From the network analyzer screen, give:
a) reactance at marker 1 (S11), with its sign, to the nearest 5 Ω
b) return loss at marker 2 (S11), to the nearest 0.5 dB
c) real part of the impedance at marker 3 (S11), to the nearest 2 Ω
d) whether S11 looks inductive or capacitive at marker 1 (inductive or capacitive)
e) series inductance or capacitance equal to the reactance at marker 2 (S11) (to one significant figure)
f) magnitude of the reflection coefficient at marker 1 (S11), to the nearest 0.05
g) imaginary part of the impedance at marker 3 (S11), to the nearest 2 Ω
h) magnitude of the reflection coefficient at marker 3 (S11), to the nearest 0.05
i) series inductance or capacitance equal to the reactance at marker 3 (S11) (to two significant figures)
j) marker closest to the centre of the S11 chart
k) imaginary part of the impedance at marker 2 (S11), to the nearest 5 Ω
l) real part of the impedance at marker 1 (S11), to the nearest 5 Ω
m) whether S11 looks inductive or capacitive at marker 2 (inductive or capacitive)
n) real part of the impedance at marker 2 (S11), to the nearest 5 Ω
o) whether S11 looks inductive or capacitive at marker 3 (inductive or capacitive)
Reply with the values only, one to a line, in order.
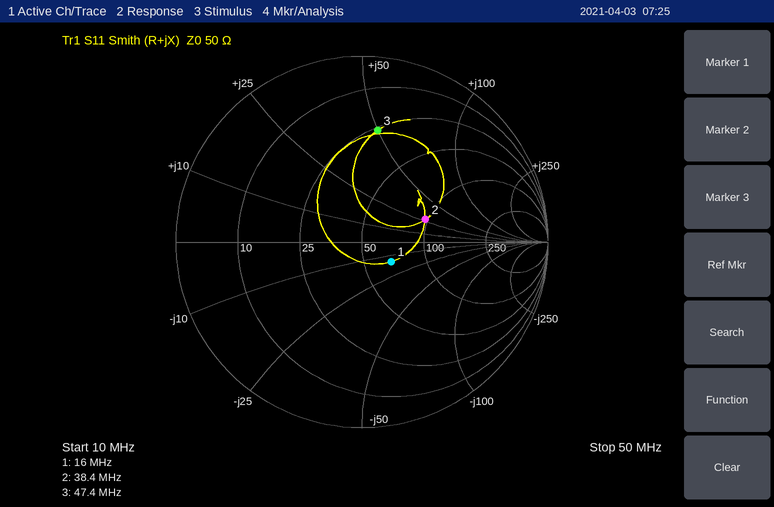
-15 Ω
9.0 dB
26 Ω
capacitive
100 nH
0.20
+50 Ω
0.60
170 nH
marker 1
+25 Ω
65 Ω
inductive
95 Ω
inductive
